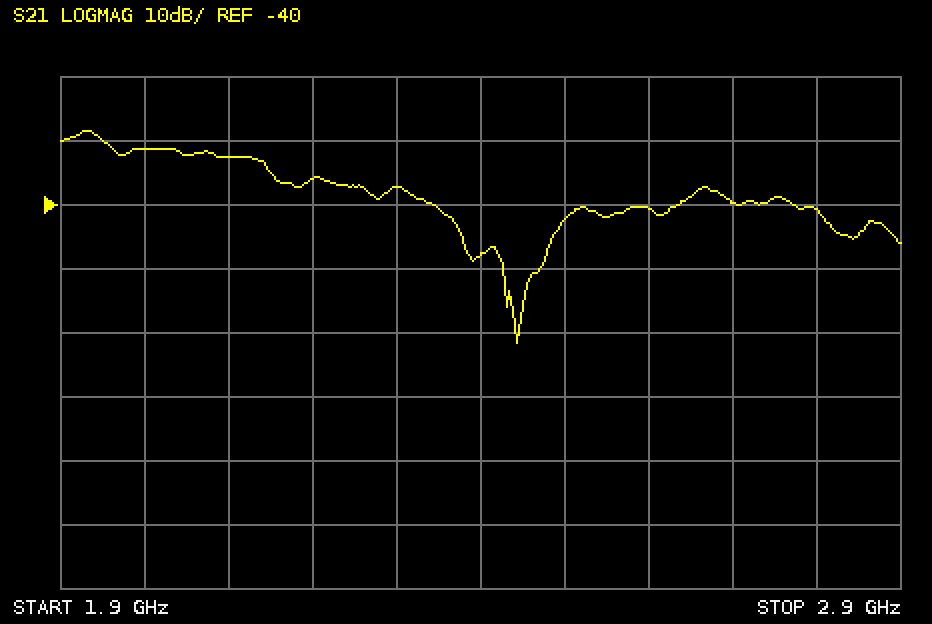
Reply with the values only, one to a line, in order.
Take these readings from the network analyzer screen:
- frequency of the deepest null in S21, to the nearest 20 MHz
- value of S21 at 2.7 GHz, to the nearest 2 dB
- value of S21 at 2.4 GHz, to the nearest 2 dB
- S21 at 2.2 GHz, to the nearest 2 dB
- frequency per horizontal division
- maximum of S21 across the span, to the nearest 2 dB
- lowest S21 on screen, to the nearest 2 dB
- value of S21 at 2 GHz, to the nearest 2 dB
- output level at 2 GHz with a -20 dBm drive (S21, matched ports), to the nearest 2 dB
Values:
2.44 GHz
-40 dB
-48 dB
-36 dB
100 MHz
-28 dB
-62 dB
-32 dB
-52 dBm
